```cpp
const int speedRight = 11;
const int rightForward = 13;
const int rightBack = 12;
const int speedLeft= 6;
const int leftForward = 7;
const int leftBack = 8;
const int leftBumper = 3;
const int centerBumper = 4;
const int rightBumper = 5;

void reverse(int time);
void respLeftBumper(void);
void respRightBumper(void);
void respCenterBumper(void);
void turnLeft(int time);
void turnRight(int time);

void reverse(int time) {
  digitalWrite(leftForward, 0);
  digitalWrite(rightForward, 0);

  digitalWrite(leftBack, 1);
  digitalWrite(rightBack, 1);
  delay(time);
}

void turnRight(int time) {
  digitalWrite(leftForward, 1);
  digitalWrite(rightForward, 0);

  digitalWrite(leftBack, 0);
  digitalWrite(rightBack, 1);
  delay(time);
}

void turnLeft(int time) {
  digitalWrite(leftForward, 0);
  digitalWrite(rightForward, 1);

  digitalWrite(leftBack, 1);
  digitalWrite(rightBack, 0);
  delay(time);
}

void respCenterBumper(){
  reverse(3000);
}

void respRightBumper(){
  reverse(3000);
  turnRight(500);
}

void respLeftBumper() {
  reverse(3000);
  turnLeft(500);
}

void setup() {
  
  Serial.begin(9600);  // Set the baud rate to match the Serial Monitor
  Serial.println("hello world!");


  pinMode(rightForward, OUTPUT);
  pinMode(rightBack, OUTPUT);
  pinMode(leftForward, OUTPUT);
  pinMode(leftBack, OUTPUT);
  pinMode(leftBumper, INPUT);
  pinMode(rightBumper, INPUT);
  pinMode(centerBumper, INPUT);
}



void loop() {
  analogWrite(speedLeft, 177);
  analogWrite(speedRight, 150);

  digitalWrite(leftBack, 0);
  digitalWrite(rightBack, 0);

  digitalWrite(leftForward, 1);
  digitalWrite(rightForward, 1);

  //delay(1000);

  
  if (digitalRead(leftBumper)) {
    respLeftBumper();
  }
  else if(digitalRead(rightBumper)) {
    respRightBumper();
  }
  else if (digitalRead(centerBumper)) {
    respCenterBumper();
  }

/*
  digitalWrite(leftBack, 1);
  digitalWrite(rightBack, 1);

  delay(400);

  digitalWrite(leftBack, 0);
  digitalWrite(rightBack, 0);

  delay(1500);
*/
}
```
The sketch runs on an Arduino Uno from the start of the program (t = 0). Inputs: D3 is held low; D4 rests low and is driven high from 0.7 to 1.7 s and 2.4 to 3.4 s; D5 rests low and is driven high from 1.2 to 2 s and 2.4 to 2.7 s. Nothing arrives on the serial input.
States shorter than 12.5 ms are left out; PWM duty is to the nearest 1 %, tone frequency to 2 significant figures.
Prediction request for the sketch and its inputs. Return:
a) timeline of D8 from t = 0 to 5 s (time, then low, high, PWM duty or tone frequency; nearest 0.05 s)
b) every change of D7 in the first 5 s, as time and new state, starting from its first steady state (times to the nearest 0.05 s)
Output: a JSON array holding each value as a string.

["0 s low; 0.7 s high; 3.7 s low", "0 s high; 0.7 s low; 3.7 s high"]
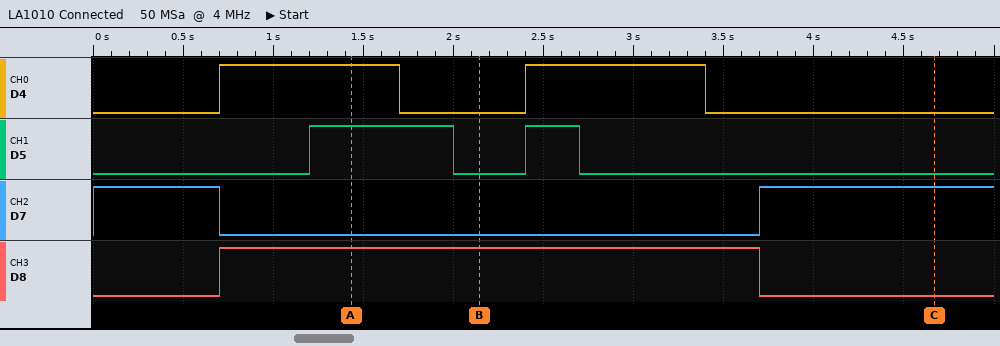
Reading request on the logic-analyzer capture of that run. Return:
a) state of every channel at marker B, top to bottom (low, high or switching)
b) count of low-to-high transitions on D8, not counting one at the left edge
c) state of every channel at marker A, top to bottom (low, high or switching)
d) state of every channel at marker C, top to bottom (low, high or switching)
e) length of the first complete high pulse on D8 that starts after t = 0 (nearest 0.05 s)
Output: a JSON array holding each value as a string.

["D4 low, D5 low, D7 low, D8 high", "1", "D4 high, D5 high, D7 low, D8 high", "D4 low, D5 low, D7 high, D8 low", "3.00 s"]
